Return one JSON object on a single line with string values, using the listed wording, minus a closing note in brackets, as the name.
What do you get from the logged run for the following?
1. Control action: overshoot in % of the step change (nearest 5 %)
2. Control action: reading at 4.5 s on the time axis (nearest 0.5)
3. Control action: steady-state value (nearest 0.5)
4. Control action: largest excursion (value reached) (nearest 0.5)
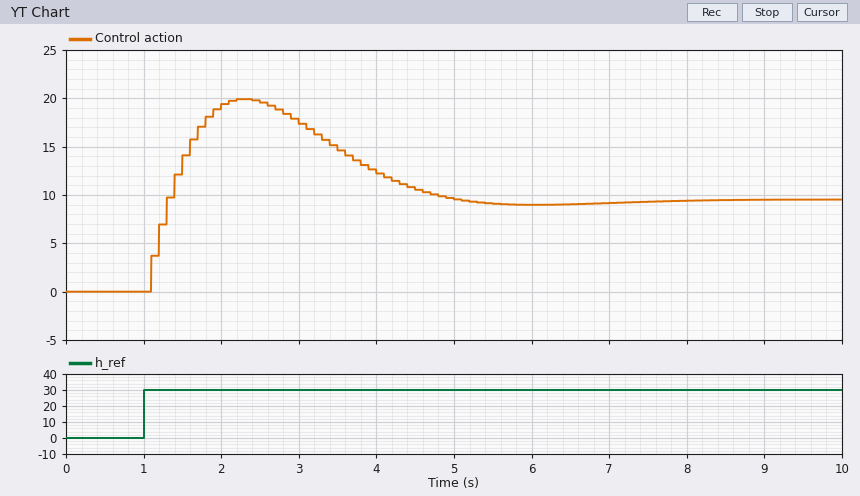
{"Control action: overshoot in % of the step change": "110 %", "Control action: reading at 4.5 s on the time axis": "10.5", "Control action: steady-state value": "9.5", "Control action: largest excursion (value reached)": "20.0"}
